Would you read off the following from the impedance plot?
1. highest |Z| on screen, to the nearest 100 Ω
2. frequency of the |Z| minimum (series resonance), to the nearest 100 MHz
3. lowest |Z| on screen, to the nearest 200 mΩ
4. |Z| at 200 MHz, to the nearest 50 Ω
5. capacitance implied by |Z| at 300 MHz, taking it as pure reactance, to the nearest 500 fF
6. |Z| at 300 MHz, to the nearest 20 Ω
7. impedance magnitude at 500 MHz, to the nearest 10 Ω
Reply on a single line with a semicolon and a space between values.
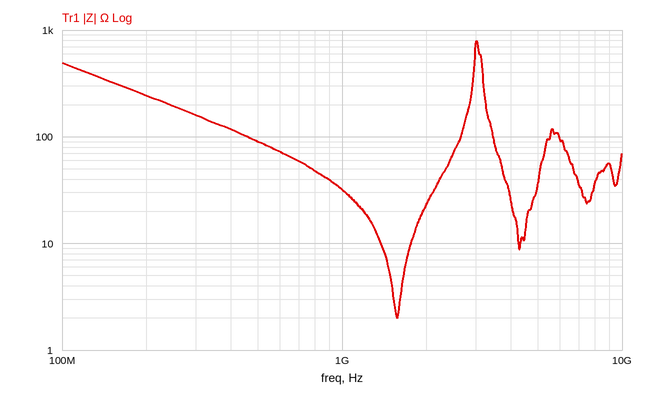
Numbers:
800 Ω; 1.6 GHz; 2.0 Ω; 250 Ω; 3.5 pF; 160 Ω; 90 Ω
